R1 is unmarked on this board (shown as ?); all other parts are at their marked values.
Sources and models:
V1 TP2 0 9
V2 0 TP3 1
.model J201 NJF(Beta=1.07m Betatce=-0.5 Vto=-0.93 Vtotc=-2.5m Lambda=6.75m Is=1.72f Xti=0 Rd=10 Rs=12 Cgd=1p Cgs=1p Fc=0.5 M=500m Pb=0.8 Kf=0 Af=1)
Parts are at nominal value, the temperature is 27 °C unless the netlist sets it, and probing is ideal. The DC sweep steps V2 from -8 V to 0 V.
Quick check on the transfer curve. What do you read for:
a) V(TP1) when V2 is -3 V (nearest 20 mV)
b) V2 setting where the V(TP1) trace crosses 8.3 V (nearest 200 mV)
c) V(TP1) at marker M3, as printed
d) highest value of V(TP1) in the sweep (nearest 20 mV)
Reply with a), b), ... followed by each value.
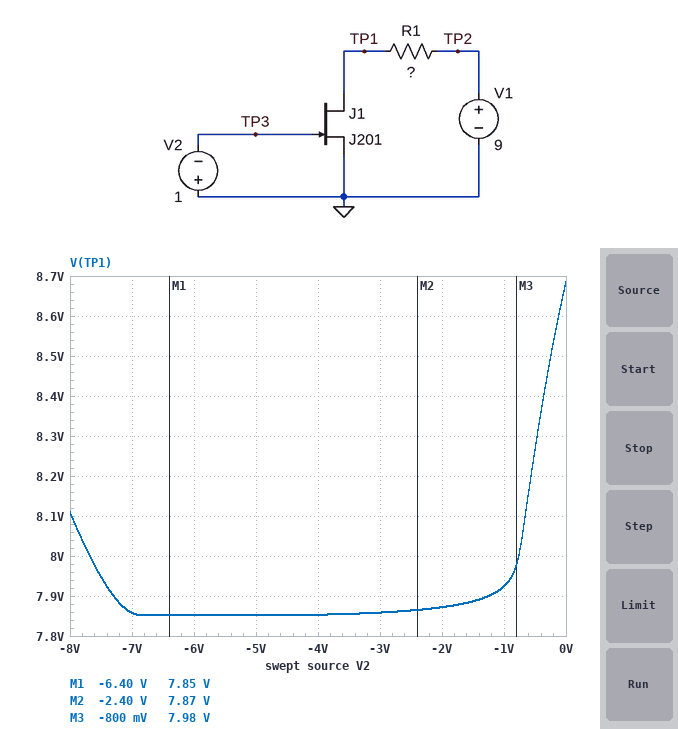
a) 7.86 V
b) -400 mV
c) 7.98 V
d) 8.68 V
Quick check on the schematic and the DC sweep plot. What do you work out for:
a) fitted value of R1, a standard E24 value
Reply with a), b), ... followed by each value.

a) 330 Ω
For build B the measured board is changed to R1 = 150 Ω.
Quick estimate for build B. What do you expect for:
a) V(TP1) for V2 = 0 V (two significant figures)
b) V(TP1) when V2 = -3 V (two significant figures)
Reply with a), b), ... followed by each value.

a) 8.9 V
b) 8.5 V
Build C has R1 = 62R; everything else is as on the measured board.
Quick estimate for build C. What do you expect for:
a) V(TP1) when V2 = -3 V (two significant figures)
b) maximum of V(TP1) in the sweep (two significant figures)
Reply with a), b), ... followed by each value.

a) 8.8 V
b) 8.9 V
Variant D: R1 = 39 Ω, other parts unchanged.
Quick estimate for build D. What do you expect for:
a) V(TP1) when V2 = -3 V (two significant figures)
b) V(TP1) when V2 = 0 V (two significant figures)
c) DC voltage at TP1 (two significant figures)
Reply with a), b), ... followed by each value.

a) 8.9 V
b) 9.0 V
c) 9.0 V
